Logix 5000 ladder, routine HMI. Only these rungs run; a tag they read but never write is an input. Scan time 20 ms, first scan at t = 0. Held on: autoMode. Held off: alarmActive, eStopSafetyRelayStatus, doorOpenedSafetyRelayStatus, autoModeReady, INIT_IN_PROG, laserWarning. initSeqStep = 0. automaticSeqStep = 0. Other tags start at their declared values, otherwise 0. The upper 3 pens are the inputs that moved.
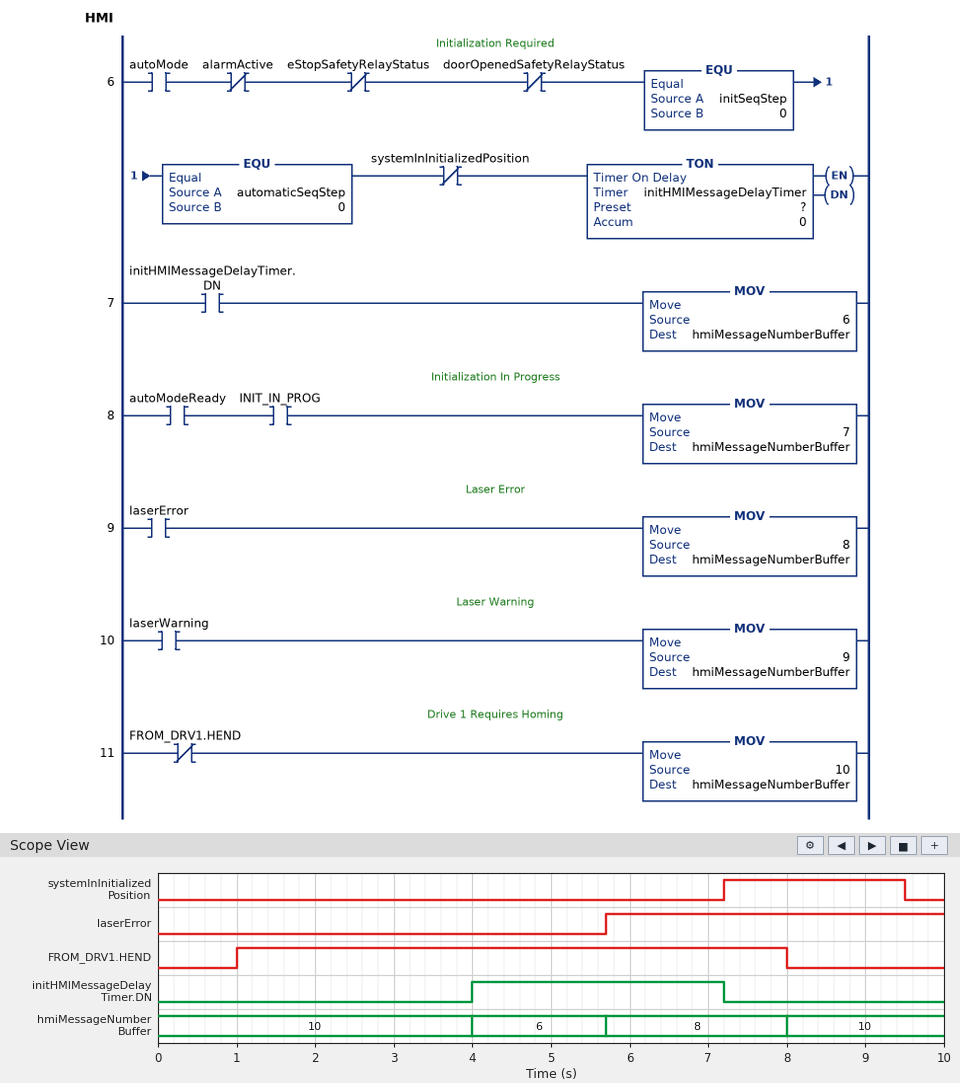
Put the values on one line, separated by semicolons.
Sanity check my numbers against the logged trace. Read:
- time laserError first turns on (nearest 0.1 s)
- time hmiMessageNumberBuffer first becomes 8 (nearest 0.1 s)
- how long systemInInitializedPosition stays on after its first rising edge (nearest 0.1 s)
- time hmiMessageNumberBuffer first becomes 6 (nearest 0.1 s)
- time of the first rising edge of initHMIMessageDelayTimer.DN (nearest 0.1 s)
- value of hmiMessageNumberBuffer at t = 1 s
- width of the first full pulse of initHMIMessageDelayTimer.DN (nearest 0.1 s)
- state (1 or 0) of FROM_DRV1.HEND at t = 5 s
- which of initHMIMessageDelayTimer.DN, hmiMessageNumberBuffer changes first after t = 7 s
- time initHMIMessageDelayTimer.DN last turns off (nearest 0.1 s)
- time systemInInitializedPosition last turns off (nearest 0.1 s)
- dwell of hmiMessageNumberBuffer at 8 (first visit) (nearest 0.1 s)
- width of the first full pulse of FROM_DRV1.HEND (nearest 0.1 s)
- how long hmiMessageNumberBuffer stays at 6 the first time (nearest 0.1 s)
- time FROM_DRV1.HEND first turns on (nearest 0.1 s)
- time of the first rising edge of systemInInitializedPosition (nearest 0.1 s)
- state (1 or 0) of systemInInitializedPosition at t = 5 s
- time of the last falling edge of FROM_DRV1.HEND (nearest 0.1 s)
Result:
5.7 s; 5.7 s; 2.3 s; 4.0 s; 4.0 s; 10; 3.2 s; 1; initHMIMessageDelayTimer.DN; 7.2 s; 9.5 s; 2.3 s; 7.0 s; 1.7 s; 1.0 s; 7.2 s; 0; 8.0 s
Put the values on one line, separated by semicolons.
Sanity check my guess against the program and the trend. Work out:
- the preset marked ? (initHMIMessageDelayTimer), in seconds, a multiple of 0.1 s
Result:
4.0 s
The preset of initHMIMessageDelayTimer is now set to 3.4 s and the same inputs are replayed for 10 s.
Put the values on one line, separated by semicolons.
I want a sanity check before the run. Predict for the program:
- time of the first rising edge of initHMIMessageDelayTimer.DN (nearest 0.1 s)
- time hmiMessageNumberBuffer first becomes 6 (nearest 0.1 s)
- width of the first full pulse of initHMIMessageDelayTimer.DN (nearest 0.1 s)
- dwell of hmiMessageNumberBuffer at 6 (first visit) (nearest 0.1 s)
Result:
3.4 s; 3.4 s; 3.8 s; 2.3 s
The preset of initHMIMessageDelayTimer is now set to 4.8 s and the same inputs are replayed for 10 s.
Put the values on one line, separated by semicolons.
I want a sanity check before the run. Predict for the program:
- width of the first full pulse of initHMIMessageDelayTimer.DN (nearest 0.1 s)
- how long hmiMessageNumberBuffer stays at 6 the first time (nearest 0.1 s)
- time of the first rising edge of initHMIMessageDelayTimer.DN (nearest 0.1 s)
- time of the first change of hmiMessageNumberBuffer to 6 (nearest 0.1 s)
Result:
2.4 s; 0.9 s; 4.8 s; 4.8 s
